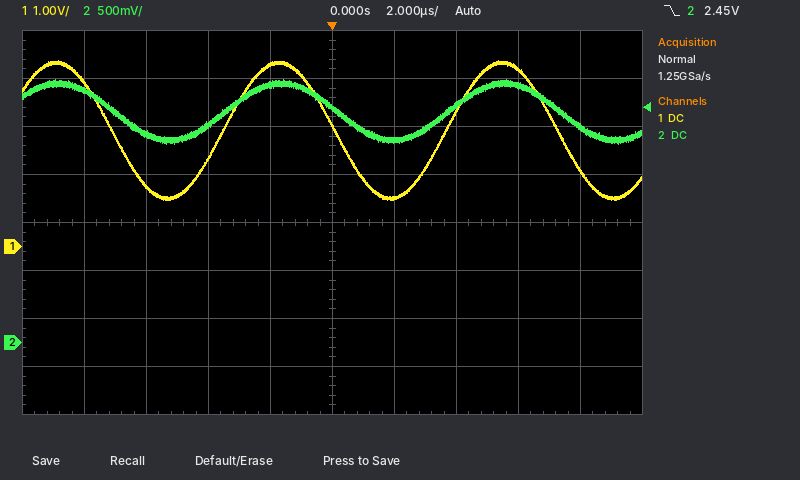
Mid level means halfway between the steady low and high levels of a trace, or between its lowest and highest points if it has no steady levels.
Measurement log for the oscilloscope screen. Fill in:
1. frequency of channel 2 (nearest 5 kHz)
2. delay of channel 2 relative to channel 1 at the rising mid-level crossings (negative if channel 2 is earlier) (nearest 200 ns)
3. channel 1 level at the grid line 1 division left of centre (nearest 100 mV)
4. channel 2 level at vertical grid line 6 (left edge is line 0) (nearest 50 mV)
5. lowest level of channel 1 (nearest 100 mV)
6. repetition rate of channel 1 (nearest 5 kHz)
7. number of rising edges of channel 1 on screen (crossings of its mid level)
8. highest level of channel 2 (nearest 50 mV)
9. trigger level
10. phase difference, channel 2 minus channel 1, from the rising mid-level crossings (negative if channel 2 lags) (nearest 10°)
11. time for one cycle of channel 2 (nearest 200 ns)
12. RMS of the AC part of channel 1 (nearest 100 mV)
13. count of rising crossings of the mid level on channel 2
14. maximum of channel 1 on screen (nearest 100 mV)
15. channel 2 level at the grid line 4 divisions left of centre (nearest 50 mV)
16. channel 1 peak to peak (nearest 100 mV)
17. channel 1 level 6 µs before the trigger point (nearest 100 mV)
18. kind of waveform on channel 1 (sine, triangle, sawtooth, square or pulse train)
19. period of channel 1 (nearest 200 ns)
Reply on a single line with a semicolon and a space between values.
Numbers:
140 kHz; 0.0 µs; 3.8 V; 2.10 V; 1.0 V; 140 kHz; 2; 2.75 V; 2.45 V; 0°; 7.2 µs; 1.0 V; 2; 3.9 V; 2.65 V; 2.9 V; 1.3 V; sine; 7.2 µs
